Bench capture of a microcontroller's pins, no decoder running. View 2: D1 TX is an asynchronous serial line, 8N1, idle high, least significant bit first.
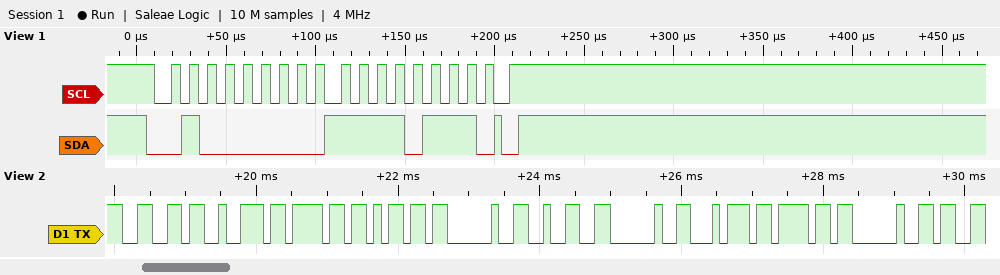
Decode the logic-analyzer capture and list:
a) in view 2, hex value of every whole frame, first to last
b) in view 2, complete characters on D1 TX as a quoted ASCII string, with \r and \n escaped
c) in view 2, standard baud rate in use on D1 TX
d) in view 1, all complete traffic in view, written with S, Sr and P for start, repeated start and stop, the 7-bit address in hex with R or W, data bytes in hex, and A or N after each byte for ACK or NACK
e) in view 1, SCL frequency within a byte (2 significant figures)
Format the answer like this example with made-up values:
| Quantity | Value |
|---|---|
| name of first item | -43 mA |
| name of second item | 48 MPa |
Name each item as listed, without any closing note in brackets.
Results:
| Quantity | Value |
|---|---|
| in view 2, hex value of every whole frame, first to last | 0x66 0x72 0x6F 0x6D 0x20 0x32 0x20 0x74 0x6F 0x20 |
| in view 2, complete characters on D1 TX as a quoted ASCII string, with \r and \n escaped | "from 2 to " |
| in view 2, standard baud rate in use on D1 TX | 9600 baud |
| in view 1, all complete traffic in view, written with S, Sr and P for start, repeated start and stop, the 7-bit address in hex with R or W, data bytes in hex, and A or N after each byte for ACK or NACK | S 20W A F7 A P |
| in view 1, SCL frequency within a byte | 100 kHz |
